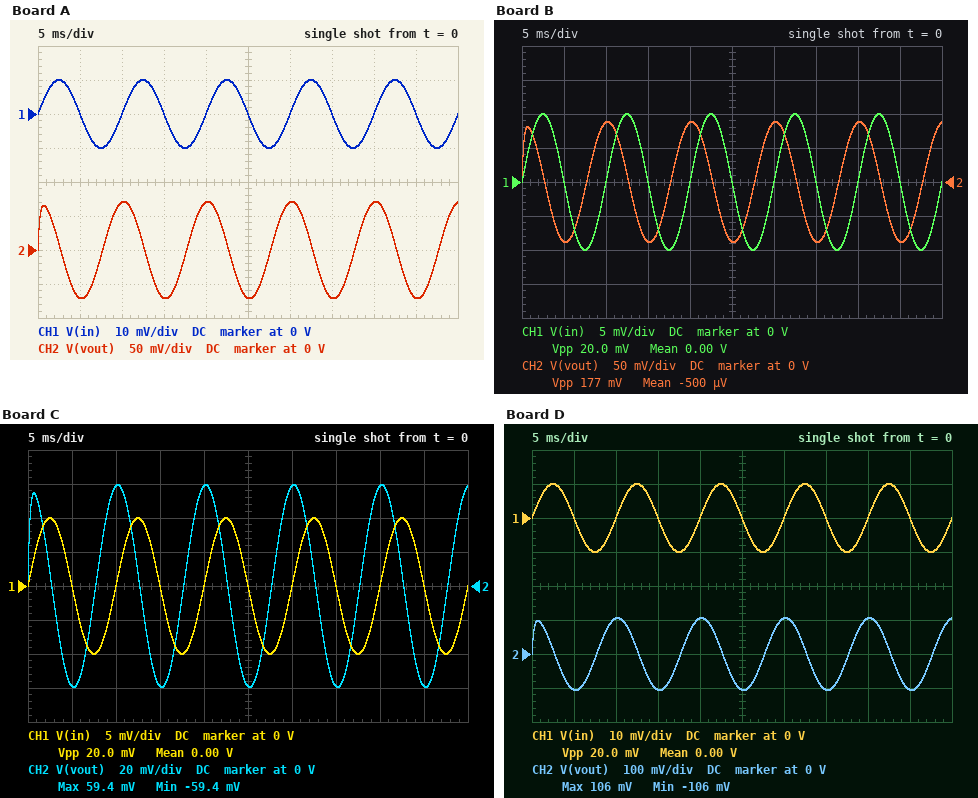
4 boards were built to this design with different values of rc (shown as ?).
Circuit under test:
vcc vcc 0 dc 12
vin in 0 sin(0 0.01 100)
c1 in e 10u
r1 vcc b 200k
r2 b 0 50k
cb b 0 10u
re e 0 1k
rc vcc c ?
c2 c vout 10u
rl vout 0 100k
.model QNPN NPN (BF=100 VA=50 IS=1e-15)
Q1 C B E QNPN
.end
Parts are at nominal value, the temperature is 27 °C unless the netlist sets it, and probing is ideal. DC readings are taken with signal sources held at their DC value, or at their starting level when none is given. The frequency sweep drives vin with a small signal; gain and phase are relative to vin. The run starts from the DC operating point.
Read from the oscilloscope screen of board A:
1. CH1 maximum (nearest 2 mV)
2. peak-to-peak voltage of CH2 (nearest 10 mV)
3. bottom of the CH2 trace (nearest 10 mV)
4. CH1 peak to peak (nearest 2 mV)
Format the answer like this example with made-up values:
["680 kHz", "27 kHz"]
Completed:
["10 mV", "140 mV", "-70 mV", "20 mV"]
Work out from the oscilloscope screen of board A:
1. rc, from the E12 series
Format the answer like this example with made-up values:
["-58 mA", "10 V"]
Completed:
["1.2 kΩ"]
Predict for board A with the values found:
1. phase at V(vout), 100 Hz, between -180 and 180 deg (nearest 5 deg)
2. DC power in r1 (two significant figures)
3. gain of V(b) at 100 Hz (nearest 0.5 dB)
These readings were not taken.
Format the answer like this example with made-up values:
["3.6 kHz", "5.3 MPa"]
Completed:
["85 deg", "500 µW", "-41.5 dB"]
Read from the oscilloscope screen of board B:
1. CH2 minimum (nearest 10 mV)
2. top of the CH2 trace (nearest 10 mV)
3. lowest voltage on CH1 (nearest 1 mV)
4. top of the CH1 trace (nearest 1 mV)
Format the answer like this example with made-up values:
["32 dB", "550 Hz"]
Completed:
["-90 mV", "90 mV", "-10 mV", "10 mV"]
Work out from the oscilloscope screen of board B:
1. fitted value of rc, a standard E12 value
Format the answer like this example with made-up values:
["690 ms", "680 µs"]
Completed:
["1.5 kΩ"]
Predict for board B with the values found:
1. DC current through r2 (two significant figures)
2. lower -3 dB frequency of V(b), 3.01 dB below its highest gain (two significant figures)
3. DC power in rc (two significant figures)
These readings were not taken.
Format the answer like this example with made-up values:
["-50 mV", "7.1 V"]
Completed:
["39 µA", "530 mHz", "2.3 mW"]
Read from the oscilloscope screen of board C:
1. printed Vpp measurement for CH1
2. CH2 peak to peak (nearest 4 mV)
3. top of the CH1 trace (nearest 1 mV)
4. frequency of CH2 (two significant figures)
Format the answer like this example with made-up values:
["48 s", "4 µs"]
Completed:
["20.0 mV", "120 mV", "10 mV", "100 Hz"]
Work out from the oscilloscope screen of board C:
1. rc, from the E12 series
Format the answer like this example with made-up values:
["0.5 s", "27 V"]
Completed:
["1 kΩ"]
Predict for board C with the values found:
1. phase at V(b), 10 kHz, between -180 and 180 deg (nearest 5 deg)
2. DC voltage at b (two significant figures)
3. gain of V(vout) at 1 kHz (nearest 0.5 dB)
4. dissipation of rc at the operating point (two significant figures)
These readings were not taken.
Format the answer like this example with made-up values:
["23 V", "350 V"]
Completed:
["-85 deg", "2.0 V", "31.5 dB", "1.6 mW"]
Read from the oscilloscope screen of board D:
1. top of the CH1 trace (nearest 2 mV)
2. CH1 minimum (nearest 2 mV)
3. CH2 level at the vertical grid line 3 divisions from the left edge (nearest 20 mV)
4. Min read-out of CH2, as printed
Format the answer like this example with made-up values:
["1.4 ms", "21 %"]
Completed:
["10 mV", "-10 mV", "-100 mV", "-106 mV"]
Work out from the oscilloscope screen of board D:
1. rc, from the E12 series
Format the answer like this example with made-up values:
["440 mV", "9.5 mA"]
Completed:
["1.8 kΩ"]
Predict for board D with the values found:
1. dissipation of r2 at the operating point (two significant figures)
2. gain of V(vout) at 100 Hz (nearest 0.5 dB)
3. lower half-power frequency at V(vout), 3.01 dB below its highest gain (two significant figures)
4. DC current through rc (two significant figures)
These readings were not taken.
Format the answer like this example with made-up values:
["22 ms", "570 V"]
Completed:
["78 µW", "20.5 dB", "770 Hz", "1.2 mA"]
